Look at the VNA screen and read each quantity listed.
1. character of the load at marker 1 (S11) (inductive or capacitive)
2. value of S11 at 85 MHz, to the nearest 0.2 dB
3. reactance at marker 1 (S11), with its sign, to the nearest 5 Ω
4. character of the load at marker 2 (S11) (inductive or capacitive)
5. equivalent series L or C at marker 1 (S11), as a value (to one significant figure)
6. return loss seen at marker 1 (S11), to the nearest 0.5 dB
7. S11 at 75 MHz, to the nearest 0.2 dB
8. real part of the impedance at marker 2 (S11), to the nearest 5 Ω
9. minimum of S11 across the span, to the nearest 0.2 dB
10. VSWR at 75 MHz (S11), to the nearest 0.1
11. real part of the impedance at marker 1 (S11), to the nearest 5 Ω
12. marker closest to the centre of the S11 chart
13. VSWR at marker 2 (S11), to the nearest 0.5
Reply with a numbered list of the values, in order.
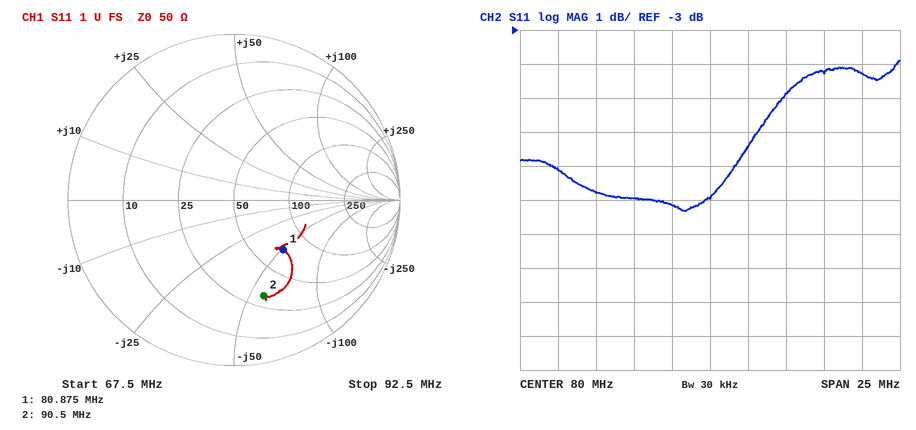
1. capacitive
2. -4.8 dB
3. -50 Ω
4. capacitive
5. 40 pF
6. 7.5 dB
7. -8.0 dB
8. 30 Ω
9. -8.4 dB
10. 2.3
11. 70 Ω
12. marker 1
13. 4.0
